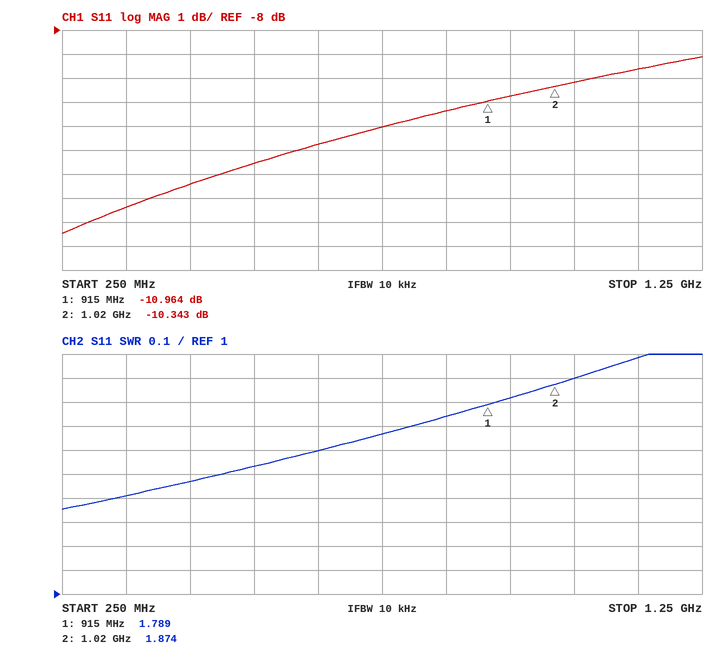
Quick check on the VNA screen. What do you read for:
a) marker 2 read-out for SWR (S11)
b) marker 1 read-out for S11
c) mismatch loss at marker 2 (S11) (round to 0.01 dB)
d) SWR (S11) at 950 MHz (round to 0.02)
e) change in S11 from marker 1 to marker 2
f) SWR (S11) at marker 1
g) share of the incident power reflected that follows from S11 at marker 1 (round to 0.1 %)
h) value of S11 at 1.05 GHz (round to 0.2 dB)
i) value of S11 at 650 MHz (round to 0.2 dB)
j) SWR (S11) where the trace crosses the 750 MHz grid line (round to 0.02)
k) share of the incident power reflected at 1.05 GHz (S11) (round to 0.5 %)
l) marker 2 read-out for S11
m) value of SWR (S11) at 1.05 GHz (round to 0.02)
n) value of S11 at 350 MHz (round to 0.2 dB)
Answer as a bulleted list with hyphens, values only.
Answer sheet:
- 1.874
- -10.964 dB
- 0.42 dB
- 1.82
- 0.621 dB
- 1.789
- 8.0 %
- -10.2 dB
- -12.8 dB
- 1.66
- 9.5 %
- -10.343 dB
- 1.90
- -15.4 dB
